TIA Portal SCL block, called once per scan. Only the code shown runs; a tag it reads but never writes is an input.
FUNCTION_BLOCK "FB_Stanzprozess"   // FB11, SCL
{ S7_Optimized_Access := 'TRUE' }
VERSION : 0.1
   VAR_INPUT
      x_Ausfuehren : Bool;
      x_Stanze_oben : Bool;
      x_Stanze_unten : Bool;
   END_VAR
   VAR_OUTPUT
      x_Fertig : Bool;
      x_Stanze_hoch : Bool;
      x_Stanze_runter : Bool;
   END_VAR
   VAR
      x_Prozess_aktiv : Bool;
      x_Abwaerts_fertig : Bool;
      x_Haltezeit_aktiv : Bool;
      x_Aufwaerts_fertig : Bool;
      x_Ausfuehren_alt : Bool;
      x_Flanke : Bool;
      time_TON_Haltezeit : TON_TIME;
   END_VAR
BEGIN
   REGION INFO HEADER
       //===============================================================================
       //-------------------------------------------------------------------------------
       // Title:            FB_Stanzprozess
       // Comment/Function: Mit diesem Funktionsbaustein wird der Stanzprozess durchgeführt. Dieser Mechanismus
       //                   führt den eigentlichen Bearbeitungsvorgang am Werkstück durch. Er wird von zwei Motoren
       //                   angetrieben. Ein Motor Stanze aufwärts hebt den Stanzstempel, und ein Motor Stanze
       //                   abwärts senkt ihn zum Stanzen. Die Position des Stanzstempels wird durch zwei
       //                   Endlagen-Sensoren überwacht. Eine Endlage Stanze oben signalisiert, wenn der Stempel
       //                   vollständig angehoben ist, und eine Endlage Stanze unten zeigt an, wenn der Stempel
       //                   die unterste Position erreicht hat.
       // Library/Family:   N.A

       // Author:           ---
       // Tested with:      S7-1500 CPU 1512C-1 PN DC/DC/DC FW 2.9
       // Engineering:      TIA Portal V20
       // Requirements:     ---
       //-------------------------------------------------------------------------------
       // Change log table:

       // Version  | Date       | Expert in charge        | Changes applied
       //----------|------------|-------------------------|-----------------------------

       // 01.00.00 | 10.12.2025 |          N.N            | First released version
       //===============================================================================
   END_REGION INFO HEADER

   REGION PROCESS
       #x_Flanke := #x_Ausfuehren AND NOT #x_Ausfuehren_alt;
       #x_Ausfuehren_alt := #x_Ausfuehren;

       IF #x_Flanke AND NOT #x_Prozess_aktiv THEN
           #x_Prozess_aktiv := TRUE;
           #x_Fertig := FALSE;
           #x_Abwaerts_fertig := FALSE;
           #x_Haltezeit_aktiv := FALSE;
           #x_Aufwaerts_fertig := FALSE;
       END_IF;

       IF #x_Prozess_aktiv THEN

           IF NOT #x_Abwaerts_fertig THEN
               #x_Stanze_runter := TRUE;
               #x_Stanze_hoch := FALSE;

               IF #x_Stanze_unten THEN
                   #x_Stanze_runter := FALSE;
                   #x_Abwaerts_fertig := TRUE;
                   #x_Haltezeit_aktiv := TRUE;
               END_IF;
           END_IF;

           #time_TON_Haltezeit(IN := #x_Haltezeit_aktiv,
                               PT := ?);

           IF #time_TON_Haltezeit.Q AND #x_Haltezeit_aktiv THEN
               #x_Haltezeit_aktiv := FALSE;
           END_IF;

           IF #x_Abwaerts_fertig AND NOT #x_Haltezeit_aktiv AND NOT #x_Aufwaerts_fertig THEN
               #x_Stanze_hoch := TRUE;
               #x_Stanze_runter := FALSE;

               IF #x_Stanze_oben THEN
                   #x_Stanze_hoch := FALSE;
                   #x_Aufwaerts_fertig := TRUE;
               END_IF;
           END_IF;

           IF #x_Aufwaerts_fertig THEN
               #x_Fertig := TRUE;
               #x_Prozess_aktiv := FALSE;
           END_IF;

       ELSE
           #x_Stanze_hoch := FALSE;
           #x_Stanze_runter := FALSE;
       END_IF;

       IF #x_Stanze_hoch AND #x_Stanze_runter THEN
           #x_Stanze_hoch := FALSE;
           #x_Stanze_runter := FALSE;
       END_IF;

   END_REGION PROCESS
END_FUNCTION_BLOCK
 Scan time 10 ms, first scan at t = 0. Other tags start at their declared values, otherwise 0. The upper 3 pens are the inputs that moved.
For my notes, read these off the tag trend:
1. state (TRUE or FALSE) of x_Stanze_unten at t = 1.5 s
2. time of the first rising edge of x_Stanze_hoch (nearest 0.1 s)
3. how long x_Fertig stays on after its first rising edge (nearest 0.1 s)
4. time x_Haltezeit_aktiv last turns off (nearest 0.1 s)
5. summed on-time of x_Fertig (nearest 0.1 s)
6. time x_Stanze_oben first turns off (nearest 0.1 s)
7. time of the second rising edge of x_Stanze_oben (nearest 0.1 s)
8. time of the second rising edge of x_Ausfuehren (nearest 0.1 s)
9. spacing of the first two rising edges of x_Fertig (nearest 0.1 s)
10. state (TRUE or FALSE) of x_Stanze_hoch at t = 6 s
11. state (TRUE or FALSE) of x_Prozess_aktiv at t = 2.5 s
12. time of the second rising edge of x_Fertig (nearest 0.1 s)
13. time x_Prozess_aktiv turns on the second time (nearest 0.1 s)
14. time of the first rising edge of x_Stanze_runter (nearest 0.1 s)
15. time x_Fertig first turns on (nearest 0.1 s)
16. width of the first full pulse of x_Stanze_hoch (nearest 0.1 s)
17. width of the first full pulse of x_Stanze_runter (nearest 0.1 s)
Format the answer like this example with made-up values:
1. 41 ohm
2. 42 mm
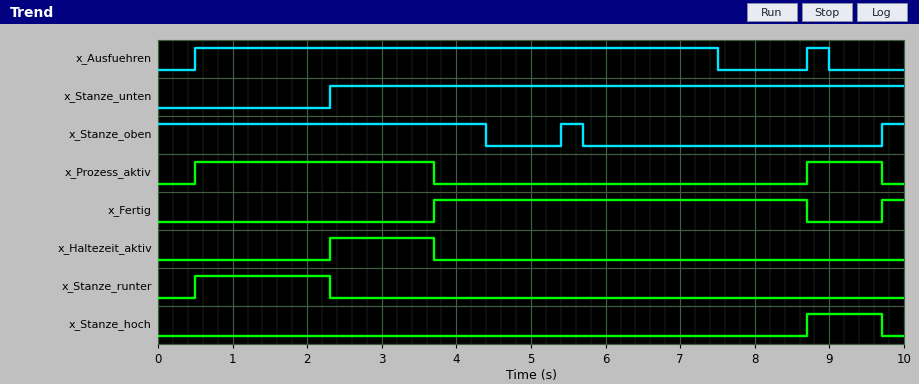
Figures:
1. FALSE
2. 8.7 s
3. 5.0 s
4. 3.7 s
5. 5.3 s
6. 4.4 s
7. 9.7 s
8. 8.7 s
9. 6.0 s
10. FALSE
11. TRUE
12. 9.7 s
13. 8.7 s
14. 0.5 s
15. 3.7 s
16. 1.0 s
17. 1.8 s
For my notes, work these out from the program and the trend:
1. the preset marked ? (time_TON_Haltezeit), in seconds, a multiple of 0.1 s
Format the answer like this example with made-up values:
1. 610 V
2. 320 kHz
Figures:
1. 1.4 s
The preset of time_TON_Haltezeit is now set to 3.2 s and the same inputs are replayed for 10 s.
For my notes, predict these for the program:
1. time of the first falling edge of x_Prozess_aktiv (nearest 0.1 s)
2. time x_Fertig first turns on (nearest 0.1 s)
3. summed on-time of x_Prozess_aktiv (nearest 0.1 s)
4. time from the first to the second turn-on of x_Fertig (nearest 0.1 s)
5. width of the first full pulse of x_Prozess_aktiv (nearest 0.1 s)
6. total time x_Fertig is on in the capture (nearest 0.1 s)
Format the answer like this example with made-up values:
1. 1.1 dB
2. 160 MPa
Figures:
1. 5.5 s
2. 5.5 s
3. 6.0 s
4. 4.2 s
5. 5.0 s
6. 3.5 s
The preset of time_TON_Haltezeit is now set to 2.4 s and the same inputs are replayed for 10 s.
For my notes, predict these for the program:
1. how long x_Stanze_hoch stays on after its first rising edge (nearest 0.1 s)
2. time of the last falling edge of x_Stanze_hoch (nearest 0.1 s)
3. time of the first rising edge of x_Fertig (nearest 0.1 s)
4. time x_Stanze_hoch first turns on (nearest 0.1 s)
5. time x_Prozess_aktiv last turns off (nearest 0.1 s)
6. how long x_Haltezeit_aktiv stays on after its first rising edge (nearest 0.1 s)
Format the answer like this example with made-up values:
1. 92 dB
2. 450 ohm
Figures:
1. 0.7 s
2. 5.4 s
3. 5.4 s
4. 4.7 s
5. 5.4 s
6. 2.4 s
